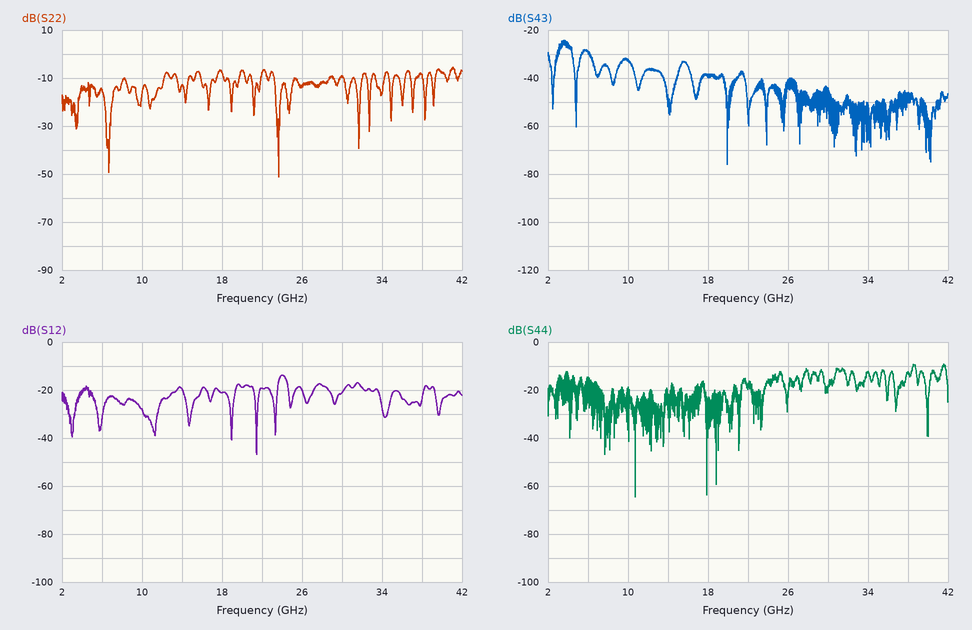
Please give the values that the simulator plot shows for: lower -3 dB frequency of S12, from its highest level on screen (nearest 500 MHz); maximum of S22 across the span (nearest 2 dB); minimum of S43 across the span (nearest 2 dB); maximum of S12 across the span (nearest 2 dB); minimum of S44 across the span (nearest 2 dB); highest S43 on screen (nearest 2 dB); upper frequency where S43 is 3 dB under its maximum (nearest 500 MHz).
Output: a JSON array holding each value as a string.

["23.5 GHz", "-6 dB", "-76 dB", "-14 dB", "-64 dB", "-24 dB", "4.0 GHz"]
